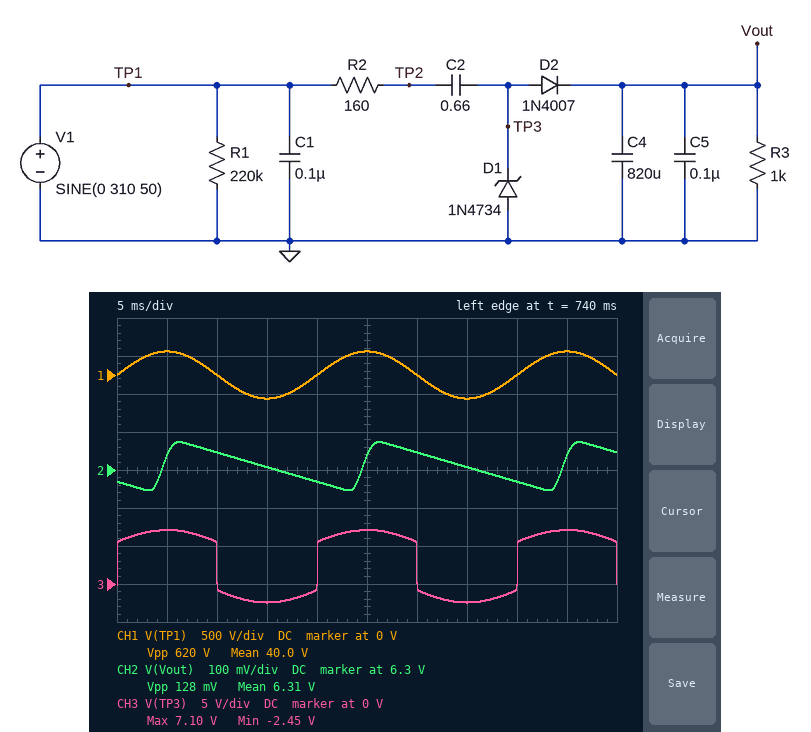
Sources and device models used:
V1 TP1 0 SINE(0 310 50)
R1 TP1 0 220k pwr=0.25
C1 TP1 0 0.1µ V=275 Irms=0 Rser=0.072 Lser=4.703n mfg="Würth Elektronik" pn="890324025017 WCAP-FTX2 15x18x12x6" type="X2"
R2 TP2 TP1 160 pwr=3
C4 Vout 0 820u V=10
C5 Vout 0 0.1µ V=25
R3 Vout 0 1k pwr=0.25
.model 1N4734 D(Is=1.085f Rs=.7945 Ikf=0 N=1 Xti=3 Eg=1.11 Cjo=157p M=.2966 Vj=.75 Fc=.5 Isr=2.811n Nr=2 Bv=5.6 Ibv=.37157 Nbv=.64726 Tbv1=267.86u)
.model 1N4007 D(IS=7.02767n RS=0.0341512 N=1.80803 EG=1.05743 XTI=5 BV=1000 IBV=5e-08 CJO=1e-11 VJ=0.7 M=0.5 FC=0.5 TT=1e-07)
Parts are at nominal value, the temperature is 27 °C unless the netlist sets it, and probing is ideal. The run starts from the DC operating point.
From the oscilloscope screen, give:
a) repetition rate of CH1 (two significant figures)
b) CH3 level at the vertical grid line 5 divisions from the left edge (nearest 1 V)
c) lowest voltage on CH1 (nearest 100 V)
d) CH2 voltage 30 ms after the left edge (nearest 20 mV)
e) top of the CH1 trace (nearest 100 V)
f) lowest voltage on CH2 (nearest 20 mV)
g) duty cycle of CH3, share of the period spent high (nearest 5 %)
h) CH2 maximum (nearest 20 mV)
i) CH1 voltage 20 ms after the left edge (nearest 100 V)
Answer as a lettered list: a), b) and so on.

a) 50 Hz
b) 7 V
c) -300 V
d) 6.34 V
e) 300 V
f) 6.24 V
g) 50 %
h) 6.38 V
i) 0 V
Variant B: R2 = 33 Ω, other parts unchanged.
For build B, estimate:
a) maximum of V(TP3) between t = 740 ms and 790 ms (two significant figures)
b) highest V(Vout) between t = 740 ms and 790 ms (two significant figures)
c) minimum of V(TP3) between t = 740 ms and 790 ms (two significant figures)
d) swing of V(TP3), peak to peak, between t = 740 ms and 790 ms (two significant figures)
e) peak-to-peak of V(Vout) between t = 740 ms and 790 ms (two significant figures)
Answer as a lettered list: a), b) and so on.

a) 13 V
b) 12 V
c) -8.2 V
d) 21 V
e) 260 mV
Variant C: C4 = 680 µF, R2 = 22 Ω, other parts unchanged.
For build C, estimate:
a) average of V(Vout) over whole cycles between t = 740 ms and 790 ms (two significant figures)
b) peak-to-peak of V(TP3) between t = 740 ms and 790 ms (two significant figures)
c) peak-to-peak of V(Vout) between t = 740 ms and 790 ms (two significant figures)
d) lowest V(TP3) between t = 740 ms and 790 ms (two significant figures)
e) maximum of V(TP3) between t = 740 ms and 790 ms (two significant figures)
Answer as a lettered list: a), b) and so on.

a) 15 V
b) 28 V
c) 410 mV
d) -12 V
e) 16 V
